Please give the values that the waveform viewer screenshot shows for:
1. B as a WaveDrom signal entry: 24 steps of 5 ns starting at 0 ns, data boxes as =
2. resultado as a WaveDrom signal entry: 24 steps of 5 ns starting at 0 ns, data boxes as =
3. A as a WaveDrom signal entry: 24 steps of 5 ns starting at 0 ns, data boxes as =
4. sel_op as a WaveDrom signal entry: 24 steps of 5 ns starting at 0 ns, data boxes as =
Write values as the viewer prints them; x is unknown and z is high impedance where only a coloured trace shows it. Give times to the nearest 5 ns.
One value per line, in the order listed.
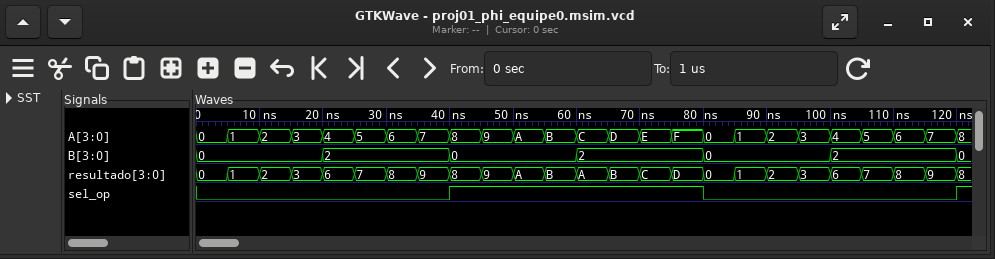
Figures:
{name: 'B', wave: '=...=...=...=...=...=...', data: '0 2 0 2 0 2'}
{name: 'resultado', wave: '========================', data: '0 1 2 3 6 7 8 9 8 9 A B A B C D 0 1 2 3 6 7 8 9'}
{name: 'A', wave: '========================', data: '0 1 2 3 4 5 6 7 8 9 A B C D E F 0 1 2 3 4 5 6 7'}
{name: 'sel_op', wave: '0.......1.......0.......'}
